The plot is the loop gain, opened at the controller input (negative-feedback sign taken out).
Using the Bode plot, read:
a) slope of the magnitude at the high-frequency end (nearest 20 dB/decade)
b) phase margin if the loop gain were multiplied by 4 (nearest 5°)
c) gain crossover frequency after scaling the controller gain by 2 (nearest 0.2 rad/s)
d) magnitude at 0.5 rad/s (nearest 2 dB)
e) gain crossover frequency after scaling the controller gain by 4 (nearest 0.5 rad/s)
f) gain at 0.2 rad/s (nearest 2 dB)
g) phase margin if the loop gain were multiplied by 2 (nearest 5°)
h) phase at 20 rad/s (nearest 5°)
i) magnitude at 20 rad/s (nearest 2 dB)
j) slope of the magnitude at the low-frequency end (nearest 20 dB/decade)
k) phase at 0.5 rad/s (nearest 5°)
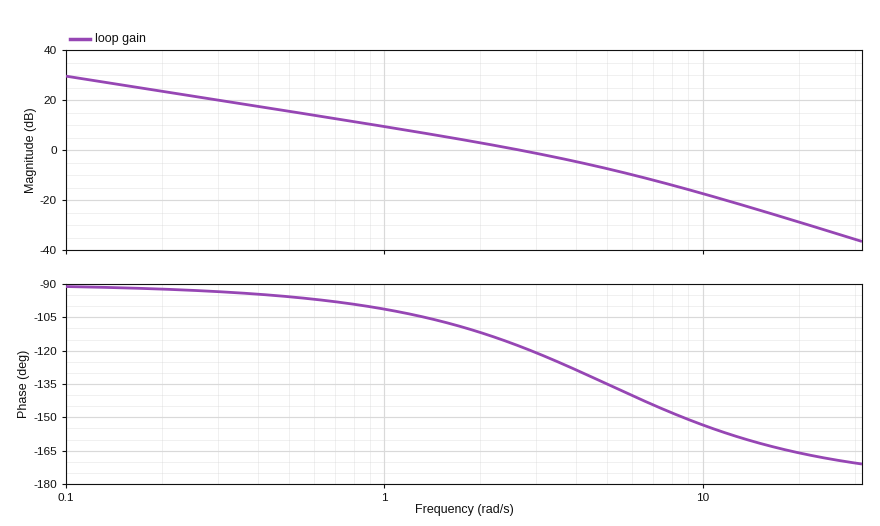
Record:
-40 dB/decade
35°
4.4 rad/s
16 dB
7.0 rad/s
24 dB
50°
-165°
-28 dB
-20 dB/decade
-95°
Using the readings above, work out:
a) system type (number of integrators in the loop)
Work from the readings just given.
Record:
1
